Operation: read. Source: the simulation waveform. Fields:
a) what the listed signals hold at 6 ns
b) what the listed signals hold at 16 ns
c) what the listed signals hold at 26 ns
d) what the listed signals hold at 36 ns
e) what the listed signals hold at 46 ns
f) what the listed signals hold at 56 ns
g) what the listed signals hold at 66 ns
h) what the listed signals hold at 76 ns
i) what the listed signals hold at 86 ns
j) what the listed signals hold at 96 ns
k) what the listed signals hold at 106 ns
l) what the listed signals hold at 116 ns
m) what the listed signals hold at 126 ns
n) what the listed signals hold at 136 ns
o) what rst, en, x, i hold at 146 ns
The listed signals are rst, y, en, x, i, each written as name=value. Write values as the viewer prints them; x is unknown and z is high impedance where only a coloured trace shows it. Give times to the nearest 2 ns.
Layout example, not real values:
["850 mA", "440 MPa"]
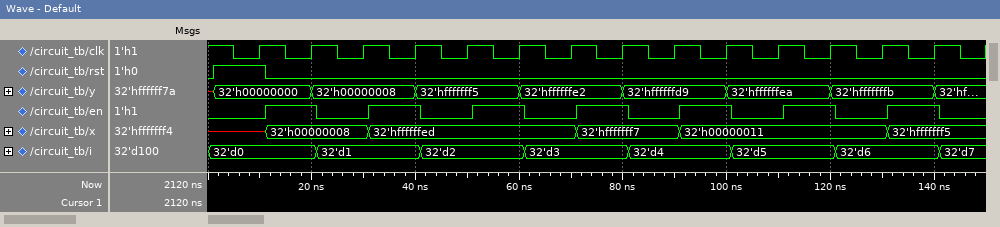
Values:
["rst=1, y=32'h00000000, en=0, x=x, i=32'd0", "rst=0, y=32'h00000000, en=1, x=32'h00000008, i=32'd0", "rst=0, y=32'h00000008, en=0, x=32'h00000008, i=32'd1", "rst=0, y=32'h00000008, en=1, x=32'hffffffed, i=32'd1", "rst=0, y=32'hfffffff5, en=0, x=32'hffffffed, i=32'd2", "rst=0, y=32'hfffffff5, en=1, x=32'hffffffed, i=32'd2", "rst=0, y=32'hffffffe2, en=0, x=32'hffffffed, i=32'd3", "rst=0, y=32'hffffffe2, en=1, x=32'hfffffff7, i=32'd3", "rst=0, y=32'hffffffd9, en=0, x=32'hfffffff7, i=32'd4", "rst=0, y=32'hffffffd9, en=1, x=32'h00000011, i=32'd4", "rst=0, y=32'hffffffea, en=0, x=32'h00000011, i=32'd5", "rst=0, y=32'hffffffea, en=1, x=32'h00000011, i=32'd5", "rst=0, y=32'hfffffffb, en=0, x=32'h00000011, i=32'd6", "rst=0, y=32'hfffffffb, en=1, x=32'hfffffff5, i=32'd6", "rst=0, en=0, x=32'hfffffff5, i=32'd7"]
